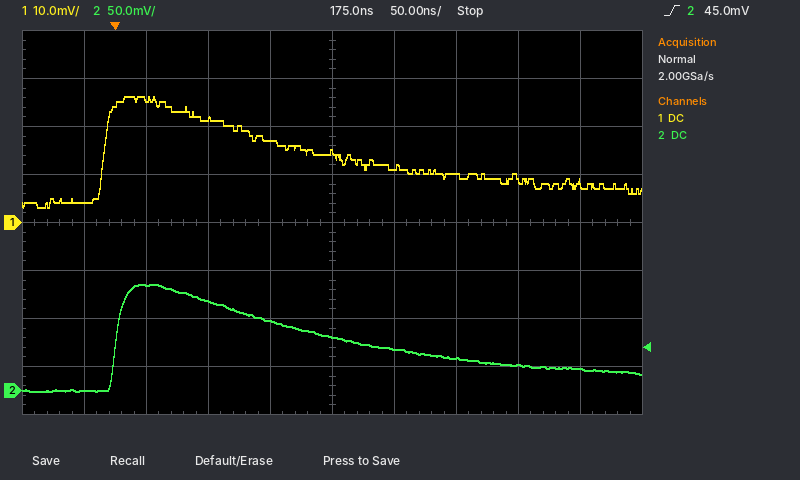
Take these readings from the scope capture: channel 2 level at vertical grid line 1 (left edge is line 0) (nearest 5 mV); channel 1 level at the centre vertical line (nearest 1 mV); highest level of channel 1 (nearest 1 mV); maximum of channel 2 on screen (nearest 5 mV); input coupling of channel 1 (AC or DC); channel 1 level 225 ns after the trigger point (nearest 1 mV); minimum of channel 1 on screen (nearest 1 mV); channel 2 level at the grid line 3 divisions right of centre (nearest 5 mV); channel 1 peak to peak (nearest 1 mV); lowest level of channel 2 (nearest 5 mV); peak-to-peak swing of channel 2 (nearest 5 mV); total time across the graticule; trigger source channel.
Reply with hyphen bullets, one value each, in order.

- 0 mV
- 15 mV
- 26 mV
- 110 mV
- DC
- 12 mV
- 3 mV
- 25 mV
- 23 mV
- 0 mV
- 110 mV
- 500 ns
- channel 2
